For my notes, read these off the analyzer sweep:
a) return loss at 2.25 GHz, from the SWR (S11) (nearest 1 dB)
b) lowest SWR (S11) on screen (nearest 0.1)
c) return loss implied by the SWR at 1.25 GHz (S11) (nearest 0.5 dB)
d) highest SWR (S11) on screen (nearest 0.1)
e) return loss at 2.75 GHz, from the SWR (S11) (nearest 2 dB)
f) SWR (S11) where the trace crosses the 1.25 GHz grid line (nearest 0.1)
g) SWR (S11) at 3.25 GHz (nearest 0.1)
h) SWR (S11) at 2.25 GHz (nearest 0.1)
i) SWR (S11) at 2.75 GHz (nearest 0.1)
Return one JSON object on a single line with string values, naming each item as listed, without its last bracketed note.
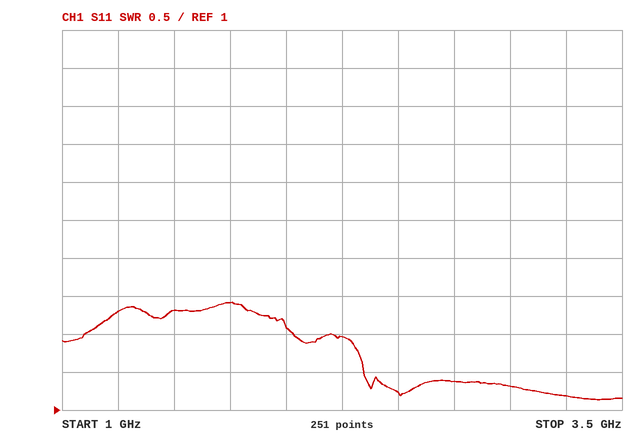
{"return loss at 2.25 GHz, from the SWR (S11)": "10 dB", "lowest SWR (S11) on screen": "1.1", "return loss implied by the SWR at 1.25 GHz (S11)": "8.0 dB", "highest SWR (S11) on screen": "2.4", "return loss at 2.75 GHz, from the SWR (S11)": "16 dB", "SWR (S11) where the trace crosses the 1.25 GHz grid line": "2.3", "SWR (S11) at 3.25 GHz": "1.2", "SWR (S11) at 2.25 GHz": "2.0", "SWR (S11) at 2.75 GHz": "1.4"}
